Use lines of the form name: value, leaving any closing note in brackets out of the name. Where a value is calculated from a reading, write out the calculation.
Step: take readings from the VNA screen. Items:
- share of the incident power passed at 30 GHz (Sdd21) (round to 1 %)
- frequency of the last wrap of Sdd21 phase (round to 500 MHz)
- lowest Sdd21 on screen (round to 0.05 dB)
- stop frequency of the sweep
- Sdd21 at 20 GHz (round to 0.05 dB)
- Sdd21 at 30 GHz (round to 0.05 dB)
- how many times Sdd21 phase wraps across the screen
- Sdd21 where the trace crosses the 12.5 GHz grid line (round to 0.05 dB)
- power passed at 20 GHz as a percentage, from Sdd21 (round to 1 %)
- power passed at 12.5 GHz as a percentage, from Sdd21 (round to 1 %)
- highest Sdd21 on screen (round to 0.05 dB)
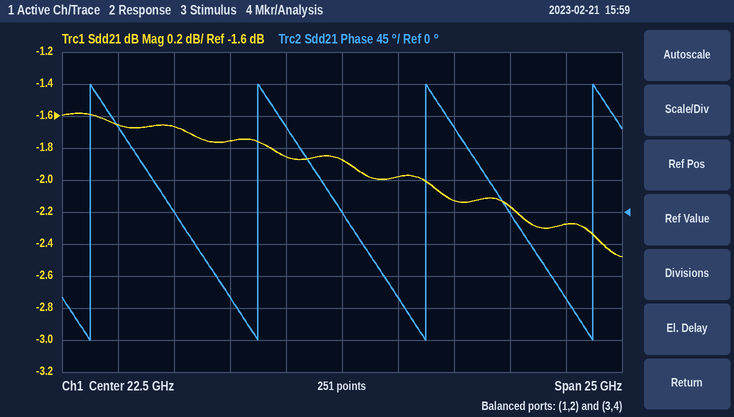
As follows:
share of the incident power passed at 30 GHz (Sdd21): 10^(-2.15/10) ≈ 61 %
frequency of the last wrap of Sdd21 phase: 33.5 GHz
lowest Sdd21 on screen: -2.50 dB
stop frequency of the sweep: 35 GHz
Sdd21 at 20 GHz: -1.85 dB
Sdd21 at 30 GHz: -2.15 dB
how many times Sdd21 phase wraps across the screen: 4
Sdd21 where the trace crosses the 12.5 GHz grid line: -1.65 dB
power passed at 20 GHz as a percentage, from Sdd21: 10^(-1.85/10) ≈ 65 %
power passed at 12.5 GHz as a percentage, from Sdd21: 10^(-1.65/10) ≈ 68 %
highest Sdd21 on screen: -1.60 dB
